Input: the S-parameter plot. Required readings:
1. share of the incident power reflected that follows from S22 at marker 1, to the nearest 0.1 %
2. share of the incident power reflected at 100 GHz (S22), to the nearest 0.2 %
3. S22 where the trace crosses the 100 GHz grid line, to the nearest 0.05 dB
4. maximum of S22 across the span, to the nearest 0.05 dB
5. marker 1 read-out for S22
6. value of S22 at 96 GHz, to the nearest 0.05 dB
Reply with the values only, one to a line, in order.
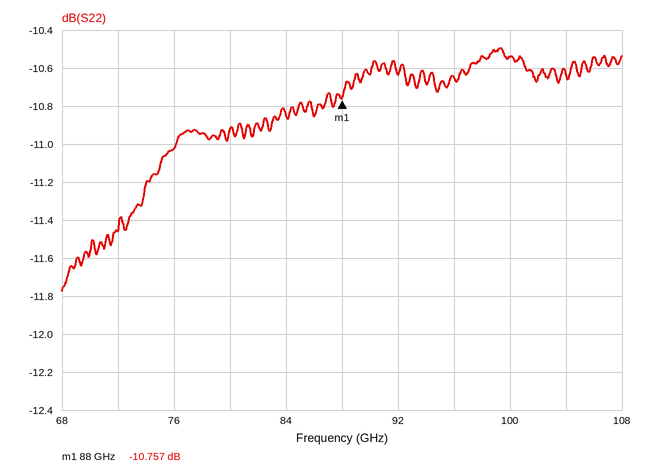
8.4 %
8.8 %
-10.55 dB
-10.50 dB
-10.757 dB
-10.65 dB
